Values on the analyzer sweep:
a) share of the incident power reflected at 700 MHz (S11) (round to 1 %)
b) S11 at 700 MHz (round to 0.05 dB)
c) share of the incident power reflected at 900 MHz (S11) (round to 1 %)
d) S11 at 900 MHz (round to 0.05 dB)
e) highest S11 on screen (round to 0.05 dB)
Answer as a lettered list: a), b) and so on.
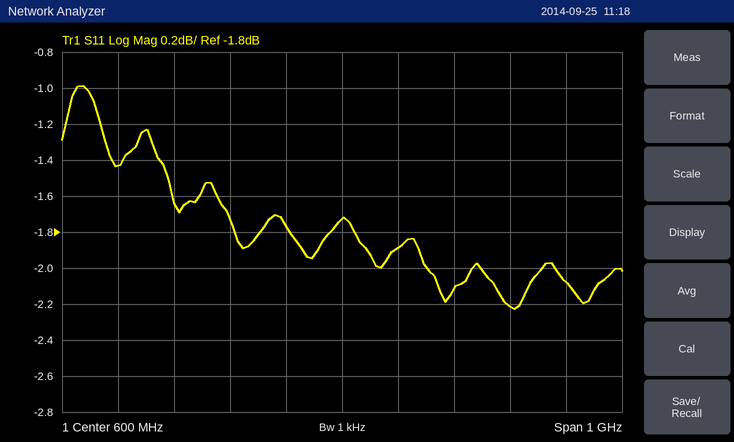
a) 65 %
b) -1.90 dB
c) 60 %
d) -2.20 dB
e) -1.00 dB
